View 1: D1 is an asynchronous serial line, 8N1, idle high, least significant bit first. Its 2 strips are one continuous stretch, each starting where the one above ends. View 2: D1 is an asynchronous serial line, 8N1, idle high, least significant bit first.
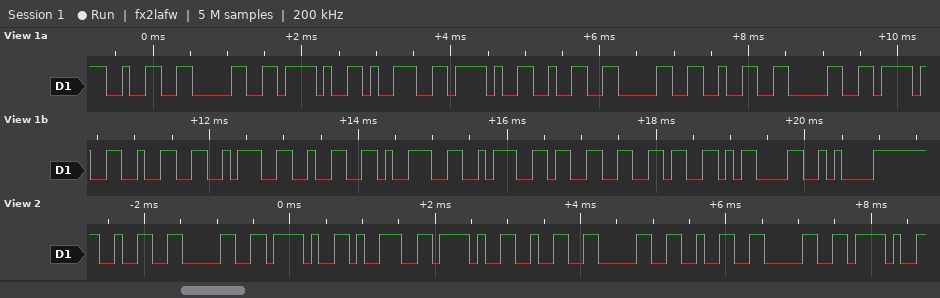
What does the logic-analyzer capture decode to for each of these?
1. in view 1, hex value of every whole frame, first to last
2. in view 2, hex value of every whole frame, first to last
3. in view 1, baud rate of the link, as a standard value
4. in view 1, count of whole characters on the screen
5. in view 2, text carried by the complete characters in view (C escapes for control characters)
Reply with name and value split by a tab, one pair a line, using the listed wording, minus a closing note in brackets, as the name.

in view 1, hex value of every whole frame, first to last	32 30 2F 39 2F 32 30 32 30 2F 32 3A 32 39 3A 33 36 0D 0A
in view 2, hex value of every whole frame, first to last	32 30 2F 39 2F 32 30 32 30 2F
in view 1, baud rate of the link, as a standard value	9600 baud
in view 1, count of whole characters on the screen	19
in view 2, text carried by the complete characters in view	"20/9/2020/"
